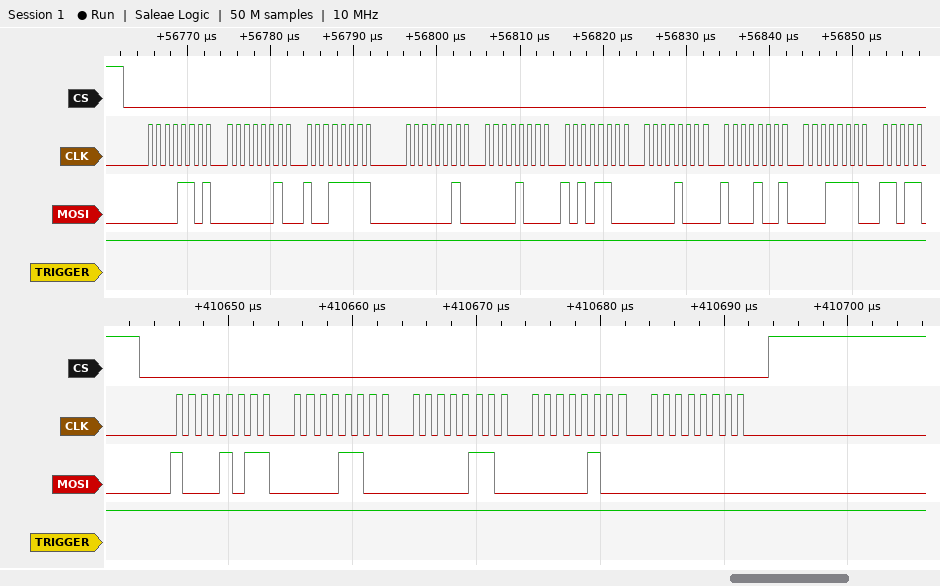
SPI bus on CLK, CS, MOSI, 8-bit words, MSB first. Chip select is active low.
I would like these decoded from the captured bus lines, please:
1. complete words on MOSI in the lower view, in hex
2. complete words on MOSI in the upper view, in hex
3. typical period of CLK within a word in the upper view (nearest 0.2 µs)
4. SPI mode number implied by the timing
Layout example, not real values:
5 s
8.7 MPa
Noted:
8B, 0C, 06, 04, 00
0D, 02, 9F, 02, 08, AC, 08, 89, 1E
1 µs
0
